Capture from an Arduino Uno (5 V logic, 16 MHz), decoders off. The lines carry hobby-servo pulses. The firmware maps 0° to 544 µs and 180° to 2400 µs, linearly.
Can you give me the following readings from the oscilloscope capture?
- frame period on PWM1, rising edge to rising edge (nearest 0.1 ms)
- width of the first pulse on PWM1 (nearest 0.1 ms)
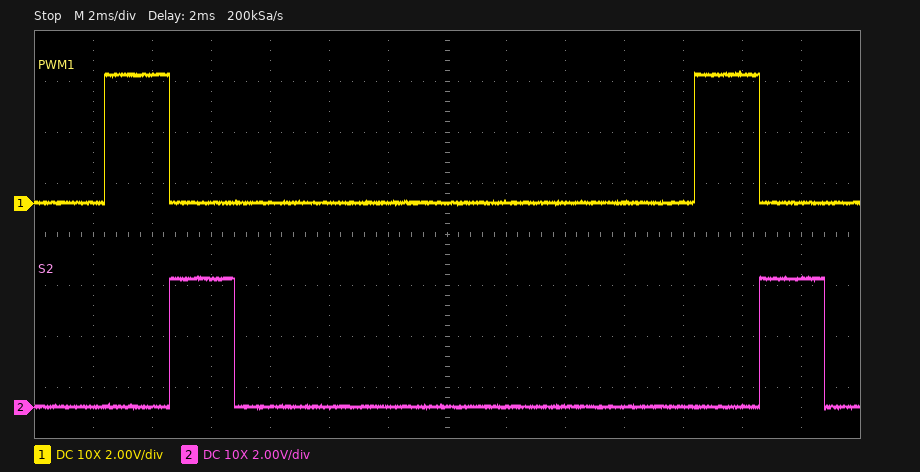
20.0 ms
2.2 ms
